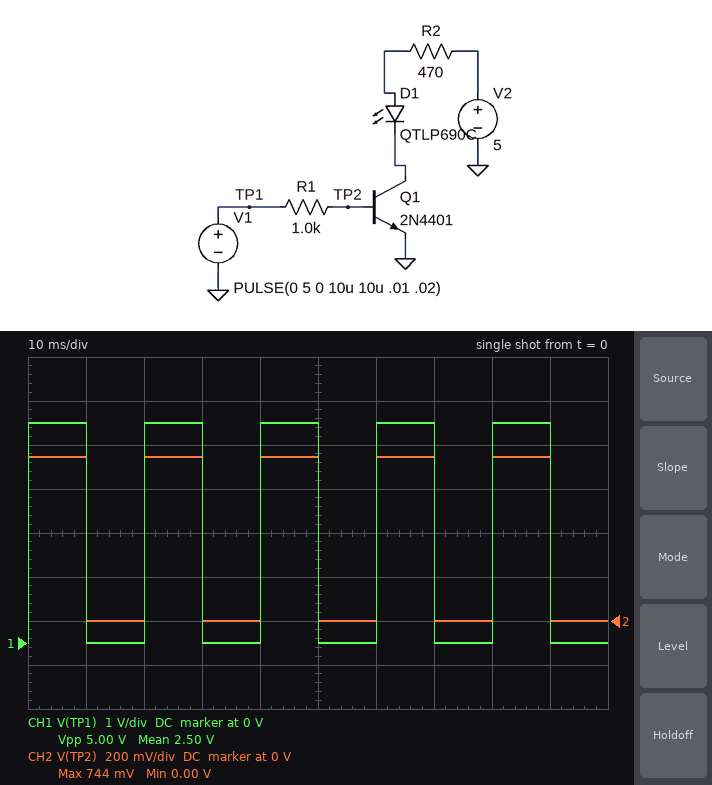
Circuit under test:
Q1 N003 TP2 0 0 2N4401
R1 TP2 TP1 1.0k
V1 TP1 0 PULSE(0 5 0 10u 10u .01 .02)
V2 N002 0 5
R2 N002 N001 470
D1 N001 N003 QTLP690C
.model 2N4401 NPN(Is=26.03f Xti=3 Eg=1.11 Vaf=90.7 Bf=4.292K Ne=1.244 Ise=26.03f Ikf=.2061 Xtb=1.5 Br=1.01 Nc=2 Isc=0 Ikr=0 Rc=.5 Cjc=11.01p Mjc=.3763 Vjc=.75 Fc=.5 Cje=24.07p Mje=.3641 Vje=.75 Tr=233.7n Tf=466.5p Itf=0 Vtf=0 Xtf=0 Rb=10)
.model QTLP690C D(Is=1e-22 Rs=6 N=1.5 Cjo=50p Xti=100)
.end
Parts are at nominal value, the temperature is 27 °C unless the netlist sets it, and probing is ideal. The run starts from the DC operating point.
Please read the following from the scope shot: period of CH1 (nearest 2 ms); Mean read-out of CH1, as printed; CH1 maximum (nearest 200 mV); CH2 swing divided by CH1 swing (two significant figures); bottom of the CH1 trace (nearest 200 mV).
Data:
20 ms
2.50 V
5.0 V
0.15
0 V
